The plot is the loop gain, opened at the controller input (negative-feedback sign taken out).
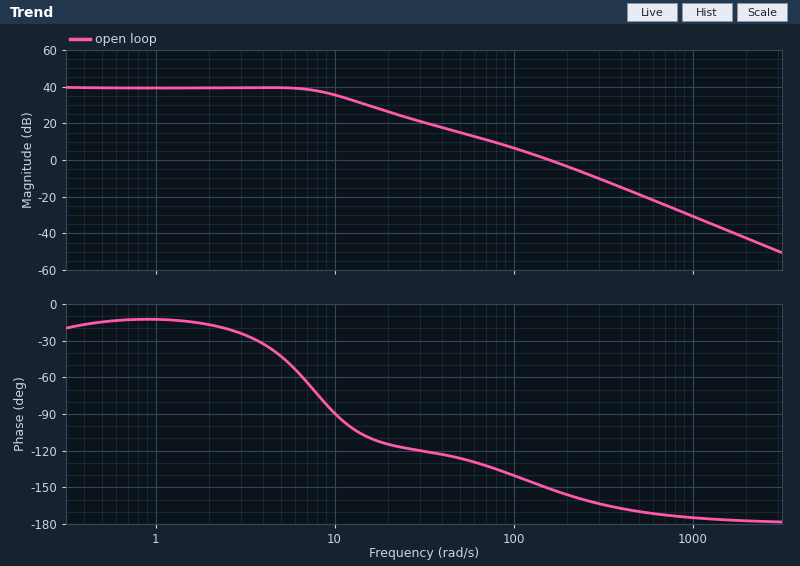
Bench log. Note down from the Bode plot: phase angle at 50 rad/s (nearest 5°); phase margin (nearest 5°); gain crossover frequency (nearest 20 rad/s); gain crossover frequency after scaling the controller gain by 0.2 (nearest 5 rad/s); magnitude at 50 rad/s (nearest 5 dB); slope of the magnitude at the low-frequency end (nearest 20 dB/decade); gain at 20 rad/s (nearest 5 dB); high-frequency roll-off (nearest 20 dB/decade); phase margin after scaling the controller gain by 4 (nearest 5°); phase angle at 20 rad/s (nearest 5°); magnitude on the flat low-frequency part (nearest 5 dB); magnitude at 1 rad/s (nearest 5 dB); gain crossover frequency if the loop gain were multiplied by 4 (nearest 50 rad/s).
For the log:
-125°
30°
160 rad/s
55 rad/s
15 dB
0 dB/decade
25 dB
-40 dB/decade
15°
-115°
40 dB
40 dB
350 rad/s
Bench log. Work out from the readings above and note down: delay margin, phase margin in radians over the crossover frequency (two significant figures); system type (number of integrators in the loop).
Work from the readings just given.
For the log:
0.0033 s
0
